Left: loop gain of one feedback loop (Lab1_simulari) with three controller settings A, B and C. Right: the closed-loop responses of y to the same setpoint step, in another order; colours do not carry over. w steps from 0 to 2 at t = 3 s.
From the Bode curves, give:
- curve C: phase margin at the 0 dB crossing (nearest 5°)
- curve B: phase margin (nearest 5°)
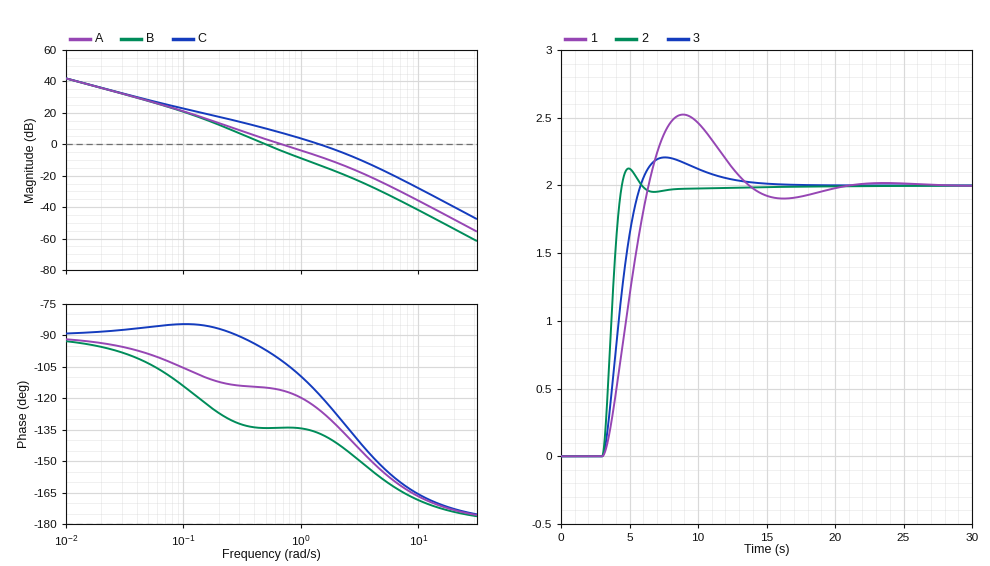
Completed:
60°
45°
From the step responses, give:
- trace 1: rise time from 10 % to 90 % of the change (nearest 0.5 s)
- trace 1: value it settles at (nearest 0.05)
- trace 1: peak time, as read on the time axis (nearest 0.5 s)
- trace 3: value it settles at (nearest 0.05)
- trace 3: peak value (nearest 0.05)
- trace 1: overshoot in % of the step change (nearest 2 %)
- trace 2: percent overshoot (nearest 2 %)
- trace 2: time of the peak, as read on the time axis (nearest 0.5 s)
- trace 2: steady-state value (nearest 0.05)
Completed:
2.5 s
2.00
9.0 s
2.00
2.20
26 %
6 %
5.0 s
2.00
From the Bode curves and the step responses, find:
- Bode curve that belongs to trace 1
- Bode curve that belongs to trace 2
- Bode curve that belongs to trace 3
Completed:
B
C
A
